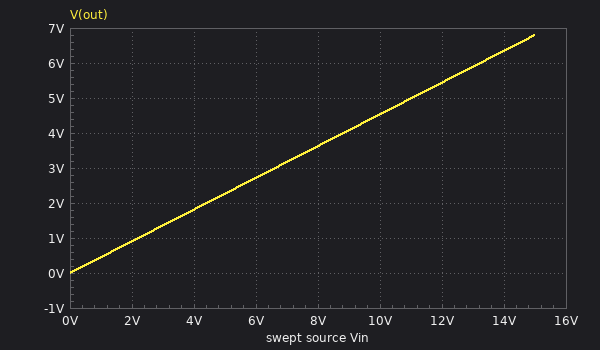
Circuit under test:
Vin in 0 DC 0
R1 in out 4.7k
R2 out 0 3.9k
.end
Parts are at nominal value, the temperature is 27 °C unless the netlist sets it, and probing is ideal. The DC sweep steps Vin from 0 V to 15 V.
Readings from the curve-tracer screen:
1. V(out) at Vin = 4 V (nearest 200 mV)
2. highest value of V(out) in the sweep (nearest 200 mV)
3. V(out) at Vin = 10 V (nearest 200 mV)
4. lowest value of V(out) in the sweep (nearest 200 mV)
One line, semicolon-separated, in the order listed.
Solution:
1.8 V; 6.8 V; 4.6 V; 0 V
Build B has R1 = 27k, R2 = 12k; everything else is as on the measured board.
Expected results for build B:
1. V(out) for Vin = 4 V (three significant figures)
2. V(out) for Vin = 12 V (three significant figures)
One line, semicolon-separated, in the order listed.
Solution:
1.23 V; 3.69 V
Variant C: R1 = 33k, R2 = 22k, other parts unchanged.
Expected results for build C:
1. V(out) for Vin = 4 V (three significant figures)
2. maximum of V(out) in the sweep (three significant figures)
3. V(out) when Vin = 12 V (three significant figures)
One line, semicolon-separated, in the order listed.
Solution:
1.60 V; 6.00 V; 4.80 V
